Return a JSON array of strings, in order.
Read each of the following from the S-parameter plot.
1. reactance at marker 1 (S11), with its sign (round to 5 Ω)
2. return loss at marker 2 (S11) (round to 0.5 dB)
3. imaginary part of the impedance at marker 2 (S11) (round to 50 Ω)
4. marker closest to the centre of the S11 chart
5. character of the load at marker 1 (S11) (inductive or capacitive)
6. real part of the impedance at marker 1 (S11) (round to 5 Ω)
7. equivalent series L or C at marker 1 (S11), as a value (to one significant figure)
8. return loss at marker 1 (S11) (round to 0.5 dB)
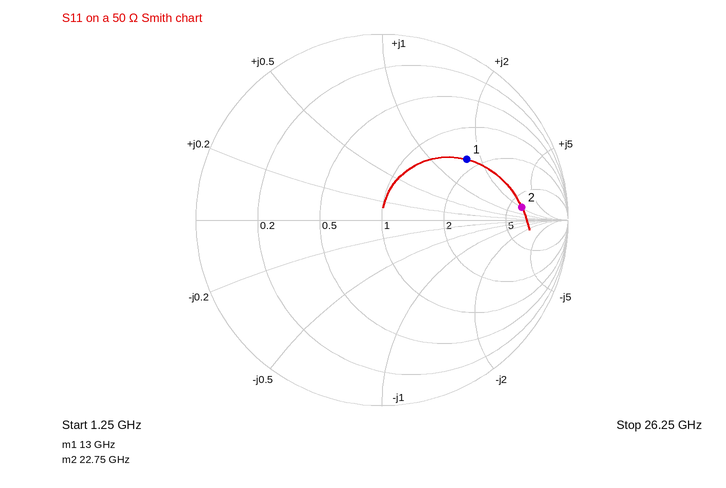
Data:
["+80 Ω", "2.5 dB", "+100 Ω", "marker 1", "inductive", "85 Ω", "1.0 nH", "5.0 dB"]
